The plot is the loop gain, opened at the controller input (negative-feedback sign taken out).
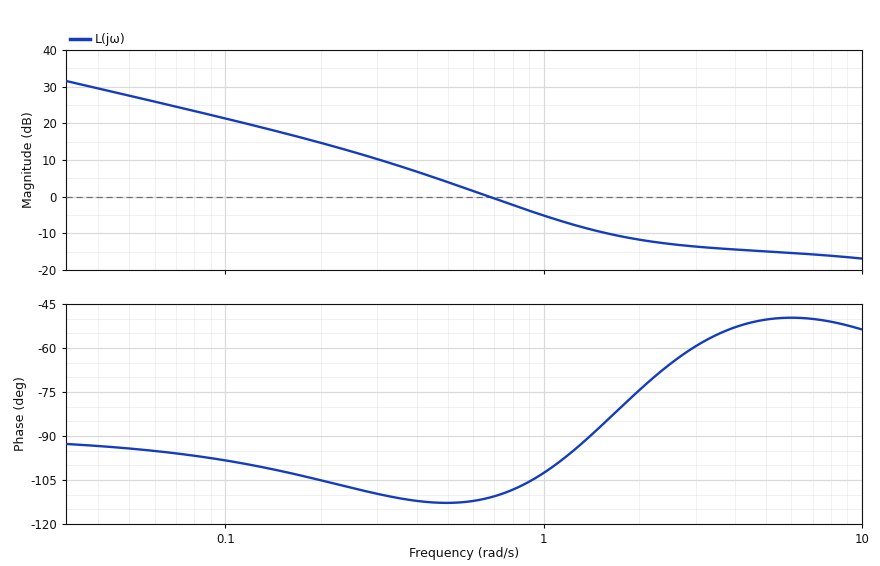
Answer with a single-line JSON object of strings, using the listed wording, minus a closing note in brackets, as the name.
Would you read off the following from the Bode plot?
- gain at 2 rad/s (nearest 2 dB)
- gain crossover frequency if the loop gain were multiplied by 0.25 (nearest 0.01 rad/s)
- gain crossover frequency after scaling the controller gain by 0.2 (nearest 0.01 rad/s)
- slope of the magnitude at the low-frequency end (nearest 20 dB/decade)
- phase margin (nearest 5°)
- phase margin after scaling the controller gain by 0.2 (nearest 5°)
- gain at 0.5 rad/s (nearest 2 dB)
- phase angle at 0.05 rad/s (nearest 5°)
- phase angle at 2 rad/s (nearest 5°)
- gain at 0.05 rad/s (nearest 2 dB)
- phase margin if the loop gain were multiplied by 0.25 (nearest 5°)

{"gain at 2 rad/s": "-12 dB", "gain crossover frequency if the loop gain were multiplied by 0.25": "0.26 rad/s", "gain crossover frequency after scaling the controller gain by 0.2": "0.21 rad/s", "slope of the magnitude at the low-frequency end": "-20 dB/decade", "phase margin": "70°", "phase margin after scaling the controller gain by 0.2": "75°", "gain at 0.5 rad/s": "4 dB", "phase angle at 0.05 rad/s": "-95°", "phase angle at 2 rad/s": "-75°", "gain at 0.05 rad/s": "28 dB", "phase margin if the loop gain were multiplied by 0.25": "70°"}
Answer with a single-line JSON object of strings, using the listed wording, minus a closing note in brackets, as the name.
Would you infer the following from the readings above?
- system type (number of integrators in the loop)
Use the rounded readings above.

{"system type": "1"}
